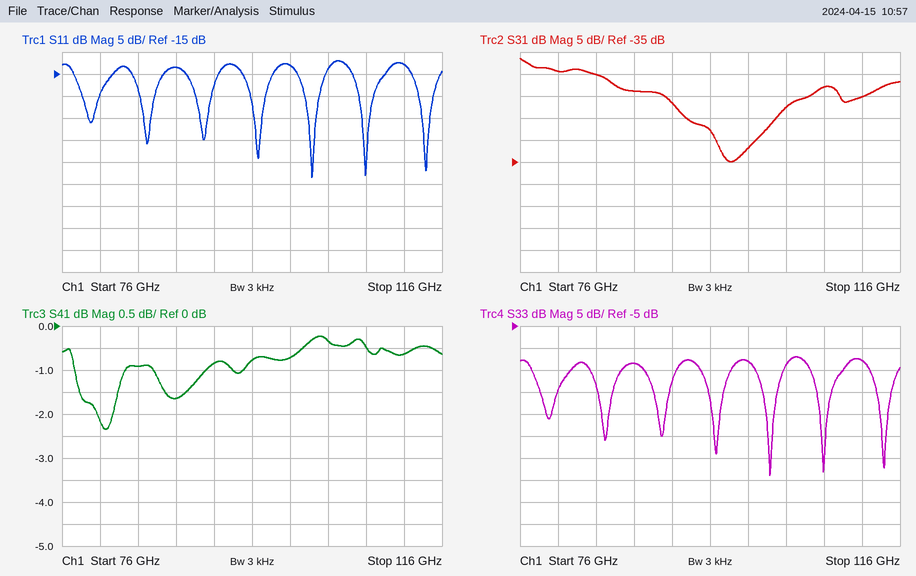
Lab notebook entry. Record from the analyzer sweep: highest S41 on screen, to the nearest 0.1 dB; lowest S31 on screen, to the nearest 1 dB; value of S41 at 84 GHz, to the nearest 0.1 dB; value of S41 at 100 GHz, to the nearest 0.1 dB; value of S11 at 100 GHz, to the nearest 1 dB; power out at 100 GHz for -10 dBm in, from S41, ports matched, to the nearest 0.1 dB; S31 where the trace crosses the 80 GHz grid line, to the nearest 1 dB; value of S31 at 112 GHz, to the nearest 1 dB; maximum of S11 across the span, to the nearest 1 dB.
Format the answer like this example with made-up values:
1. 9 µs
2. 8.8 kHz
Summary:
1. -0.2 dB
2. -35 dB
3. -0.9 dB
4. -0.7 dB
5. -13 dB
6. -10.7 dBm
7. -14 dB
8. -20 dB
9. -12 dB
